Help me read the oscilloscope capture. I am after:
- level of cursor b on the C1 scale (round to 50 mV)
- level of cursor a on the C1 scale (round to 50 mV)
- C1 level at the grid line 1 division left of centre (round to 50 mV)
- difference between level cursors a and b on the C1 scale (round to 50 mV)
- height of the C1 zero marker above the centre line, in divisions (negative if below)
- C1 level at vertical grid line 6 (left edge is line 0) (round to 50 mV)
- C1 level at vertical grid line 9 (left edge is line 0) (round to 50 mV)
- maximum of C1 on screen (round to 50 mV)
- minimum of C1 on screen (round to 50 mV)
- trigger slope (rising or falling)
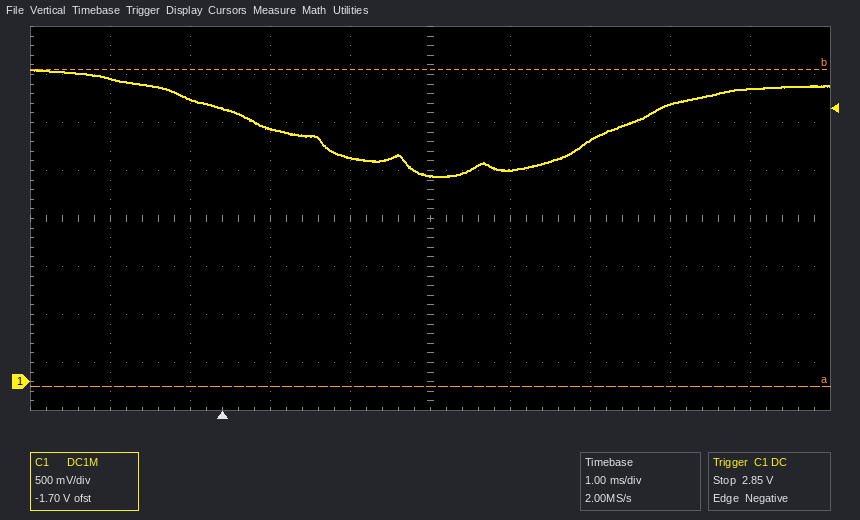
3.25 V
-50 mV
2.35 V
3.30 V
-3.4 div
2.20 V
3.05 V
3.25 V
2.15 V
falling
